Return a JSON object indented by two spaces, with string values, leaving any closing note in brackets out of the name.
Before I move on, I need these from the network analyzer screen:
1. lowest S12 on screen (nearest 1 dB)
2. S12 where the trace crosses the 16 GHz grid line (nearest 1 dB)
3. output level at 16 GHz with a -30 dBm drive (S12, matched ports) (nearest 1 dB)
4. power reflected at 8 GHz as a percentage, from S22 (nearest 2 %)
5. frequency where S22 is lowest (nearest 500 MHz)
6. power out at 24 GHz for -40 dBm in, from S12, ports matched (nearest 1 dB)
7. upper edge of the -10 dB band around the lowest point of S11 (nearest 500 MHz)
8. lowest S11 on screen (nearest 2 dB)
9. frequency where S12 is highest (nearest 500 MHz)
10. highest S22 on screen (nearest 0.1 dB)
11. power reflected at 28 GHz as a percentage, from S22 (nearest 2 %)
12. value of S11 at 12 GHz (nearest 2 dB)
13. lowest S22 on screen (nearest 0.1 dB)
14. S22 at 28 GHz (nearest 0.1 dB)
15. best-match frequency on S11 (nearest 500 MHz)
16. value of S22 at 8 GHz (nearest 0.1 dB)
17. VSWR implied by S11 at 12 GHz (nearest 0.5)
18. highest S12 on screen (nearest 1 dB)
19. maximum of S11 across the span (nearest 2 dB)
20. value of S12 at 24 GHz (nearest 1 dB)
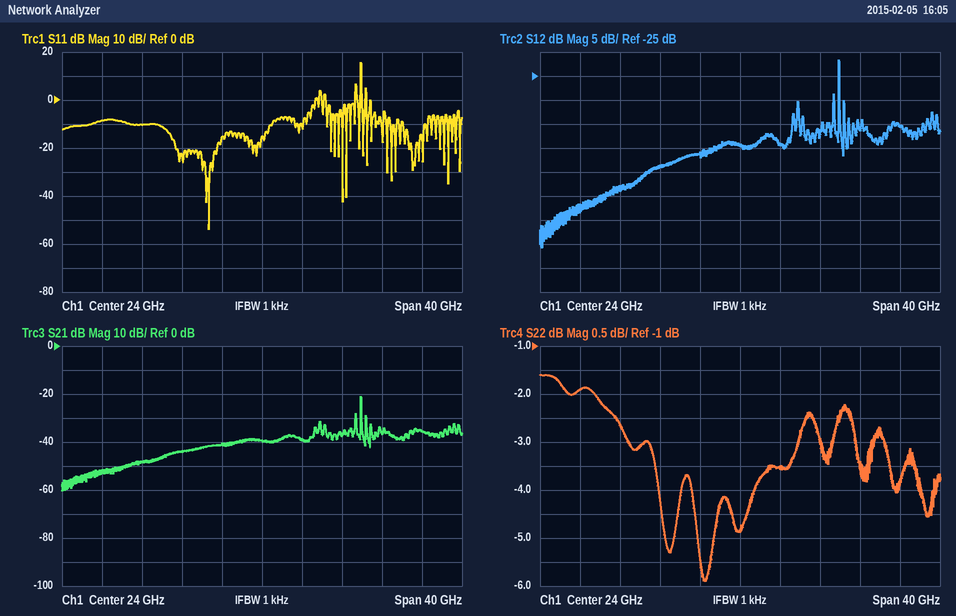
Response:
{
  "lowest S12 on screen": "-61 dB",
  "S12 where the trace crosses the 16 GHz grid line": "-44 dB",
  "output level at 16 GHz with a -30 dBm drive (S12, matched ports)": "-74 dBm",
  "power reflected at 8 GHz as a percentage, from S22": "64 %",
  "frequency where S22 is lowest": "20.5 GHz",
  "power out at 24 GHz for -40 dBm in, from S12, ports matched": "-79 dBm",
  "upper edge of the -10 dB band around the lowest point of S11": "25.0 GHz",
  "lowest S11 on screen": "-54 dB",
  "frequency where S12 is highest": "34.0 GHz",
  "highest S22 on screen": "-1.6 dB",
  "power reflected at 28 GHz as a percentage, from S22": "44 %",
  "value of S11 at 12 GHz": "-10 dB",
  "lowest S22 on screen": "-5.9 dB",
  "S22 at 28 GHz": "-3.5 dB",
  "best-match frequency on S11": "18.5 GHz",
  "value of S22 at 8 GHz": "-1.9 dB",
  "VSWR implied by S11 at 12 GHz": "2.0",
  "highest S12 on screen": "-22 dB",
  "maximum of S11 across the span": "16 dB",
  "value of S12 at 24 GHz": "-39 dB"
}
